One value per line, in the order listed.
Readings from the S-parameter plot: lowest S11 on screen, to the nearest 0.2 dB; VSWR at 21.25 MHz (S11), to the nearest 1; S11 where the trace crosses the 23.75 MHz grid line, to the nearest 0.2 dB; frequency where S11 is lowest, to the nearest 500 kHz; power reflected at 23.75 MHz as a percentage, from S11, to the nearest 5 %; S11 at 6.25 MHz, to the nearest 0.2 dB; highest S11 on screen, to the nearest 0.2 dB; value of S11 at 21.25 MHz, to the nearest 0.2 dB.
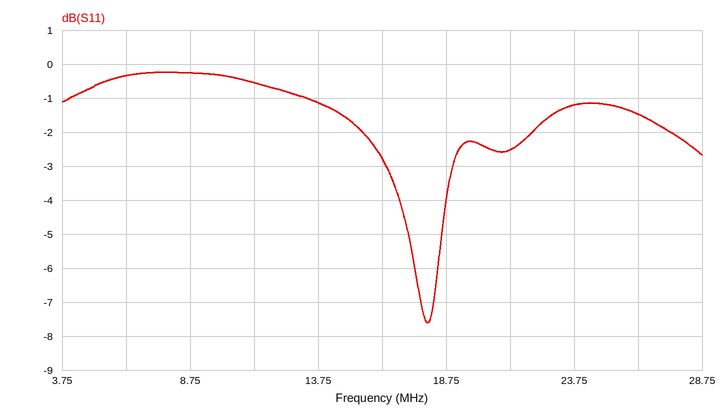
-7.6 dB
7
-1.2 dB
18.0 MHz
75 %
-0.4 dB
-0.2 dB
-2.6 dB
